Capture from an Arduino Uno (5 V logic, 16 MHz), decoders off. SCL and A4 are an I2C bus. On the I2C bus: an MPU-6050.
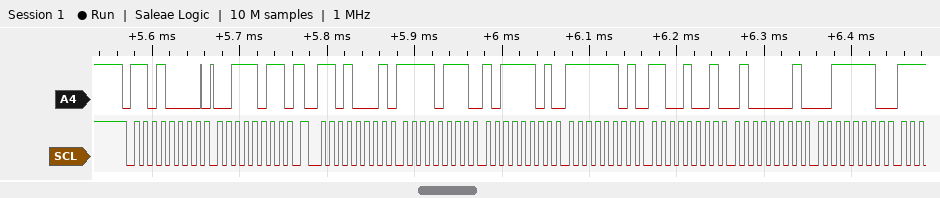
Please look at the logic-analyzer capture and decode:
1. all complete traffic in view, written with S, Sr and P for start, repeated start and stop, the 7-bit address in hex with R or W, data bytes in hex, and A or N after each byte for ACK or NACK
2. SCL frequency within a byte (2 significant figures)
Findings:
S 68W A 3B A Sr 68R A F7 A BD A FD A C9 A 41 A 3E A
100 kHz
